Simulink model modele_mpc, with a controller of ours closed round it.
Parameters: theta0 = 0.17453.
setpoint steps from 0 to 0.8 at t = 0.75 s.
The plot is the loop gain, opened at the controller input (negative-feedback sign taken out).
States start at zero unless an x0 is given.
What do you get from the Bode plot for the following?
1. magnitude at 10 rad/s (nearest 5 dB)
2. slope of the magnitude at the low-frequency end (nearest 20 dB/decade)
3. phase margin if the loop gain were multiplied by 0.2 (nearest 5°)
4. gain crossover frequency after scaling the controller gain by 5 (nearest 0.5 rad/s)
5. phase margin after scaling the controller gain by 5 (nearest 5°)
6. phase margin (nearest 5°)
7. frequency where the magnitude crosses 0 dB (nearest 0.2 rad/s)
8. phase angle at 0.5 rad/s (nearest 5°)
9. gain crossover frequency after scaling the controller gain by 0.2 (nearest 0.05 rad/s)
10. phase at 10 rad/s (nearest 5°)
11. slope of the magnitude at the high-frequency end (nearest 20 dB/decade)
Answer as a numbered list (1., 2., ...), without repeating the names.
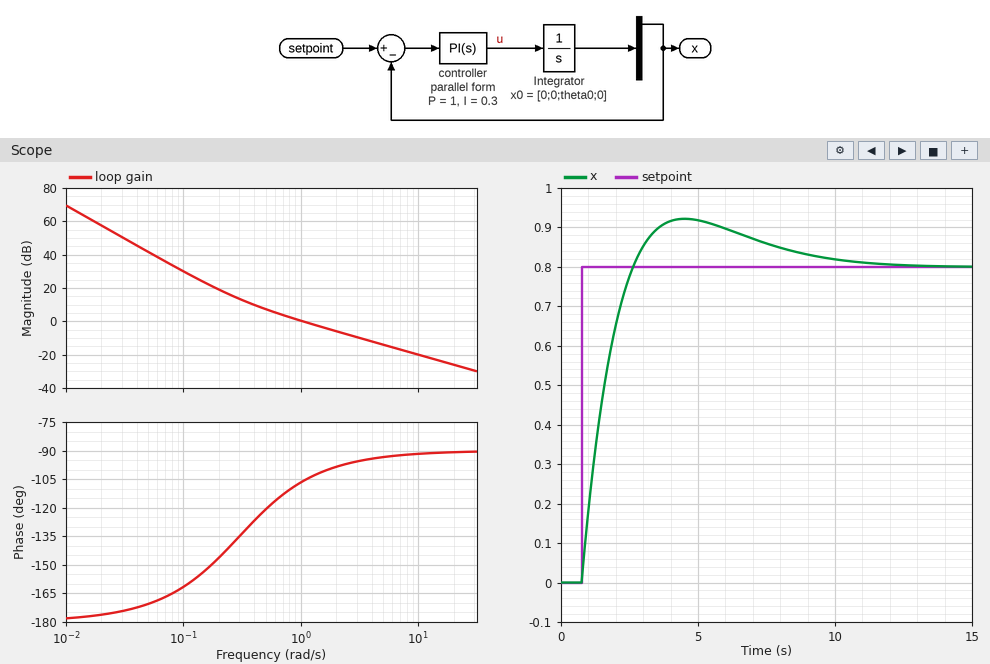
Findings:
1. -20 dB
2. -40 dB/decade
3. 45°
4. 5.0 rad/s
5. 85°
6. 75°
7. 1.0 rad/s
8. -120°
9. 0.30 rad/s
10. -90°
11. -20 dB/decade
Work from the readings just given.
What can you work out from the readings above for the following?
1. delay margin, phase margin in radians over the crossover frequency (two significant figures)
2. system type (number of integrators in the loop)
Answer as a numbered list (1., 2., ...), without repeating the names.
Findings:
1. 1.3 s
2. 2
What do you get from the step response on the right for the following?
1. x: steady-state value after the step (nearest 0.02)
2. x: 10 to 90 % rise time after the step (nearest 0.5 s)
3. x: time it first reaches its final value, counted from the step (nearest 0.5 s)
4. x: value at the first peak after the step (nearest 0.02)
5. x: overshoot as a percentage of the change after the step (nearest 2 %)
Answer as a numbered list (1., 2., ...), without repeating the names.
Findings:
1. 0.80
2. 1.5 s
3. 2.0 s
4. 0.92
5. 16 %
